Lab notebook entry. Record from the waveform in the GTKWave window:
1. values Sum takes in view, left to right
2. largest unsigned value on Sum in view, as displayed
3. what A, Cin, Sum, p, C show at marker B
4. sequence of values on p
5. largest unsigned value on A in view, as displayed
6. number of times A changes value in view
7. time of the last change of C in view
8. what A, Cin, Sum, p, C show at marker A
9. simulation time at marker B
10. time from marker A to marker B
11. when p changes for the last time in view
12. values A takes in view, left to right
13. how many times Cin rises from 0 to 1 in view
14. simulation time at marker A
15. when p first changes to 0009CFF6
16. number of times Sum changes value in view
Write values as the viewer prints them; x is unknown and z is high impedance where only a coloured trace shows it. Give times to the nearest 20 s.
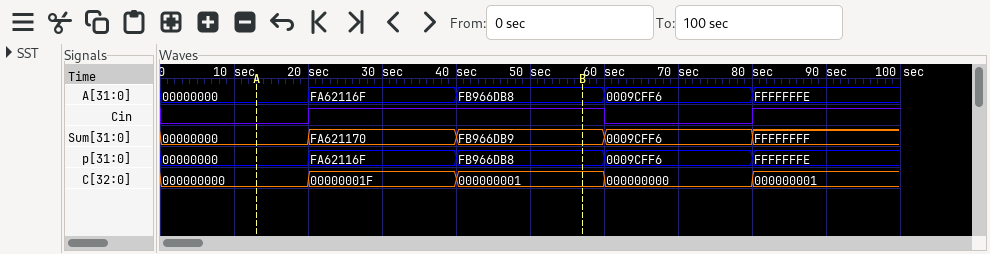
00000000, FA621170, FB966DB9, 0009CFF6, FFFFFFFF
FFFFFFFF
A=FB966DB8, Cin=1, Sum=FB966DB9, p=FB966DB8, C=000000001
00000000, FA62116F, FB966DB8, 0009CFF6, FFFFFFFE
FFFFFFFE
4
80 s
A=00000000, Cin=0, Sum=00000000, p=00000000, C=000000000
60 s
40 s
80 s
00000000, FA62116F, FB966DB8, 0009CFF6, FFFFFFFE
2
20 s
60 s
4
